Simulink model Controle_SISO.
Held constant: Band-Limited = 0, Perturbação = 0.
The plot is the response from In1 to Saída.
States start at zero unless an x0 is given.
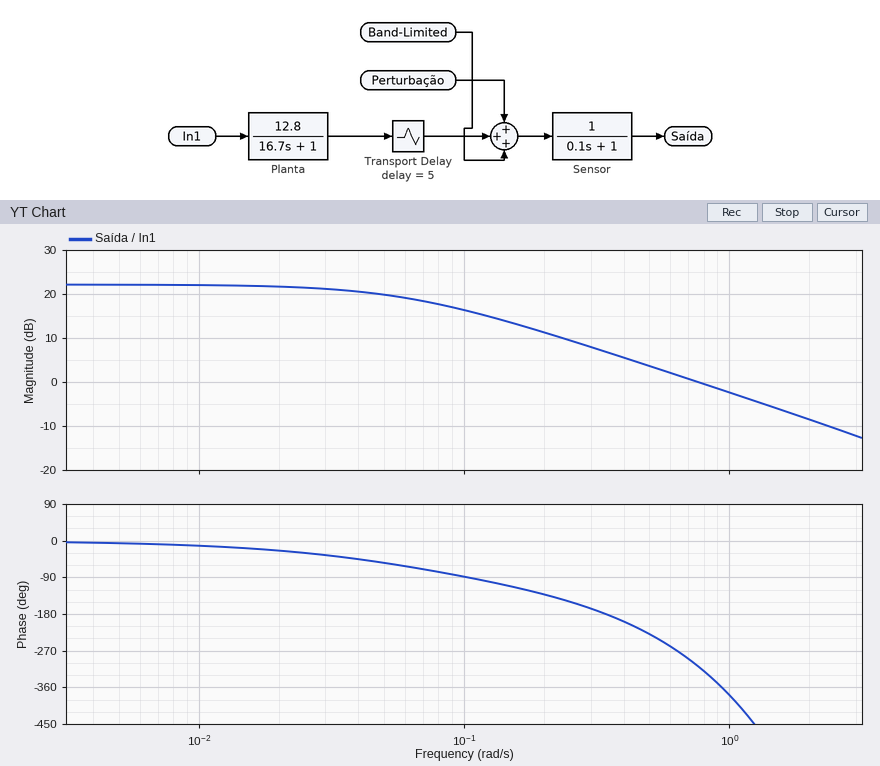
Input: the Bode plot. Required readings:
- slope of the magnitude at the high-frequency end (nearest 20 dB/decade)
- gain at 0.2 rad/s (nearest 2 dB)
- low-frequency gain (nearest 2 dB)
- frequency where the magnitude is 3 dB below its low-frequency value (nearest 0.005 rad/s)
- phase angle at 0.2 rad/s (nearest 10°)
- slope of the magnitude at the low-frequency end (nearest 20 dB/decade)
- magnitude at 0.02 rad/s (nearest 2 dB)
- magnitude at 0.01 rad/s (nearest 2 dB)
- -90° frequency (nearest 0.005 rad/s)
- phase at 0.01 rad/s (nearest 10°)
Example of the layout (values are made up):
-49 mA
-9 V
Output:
-20 dB/decade
12 dB
22 dB
0.060 rad/s
-130°
0 dB/decade
22 dB
22 dB
0.105 rad/s
-10°
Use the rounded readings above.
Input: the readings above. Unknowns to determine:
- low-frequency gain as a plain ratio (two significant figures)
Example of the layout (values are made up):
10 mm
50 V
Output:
13
